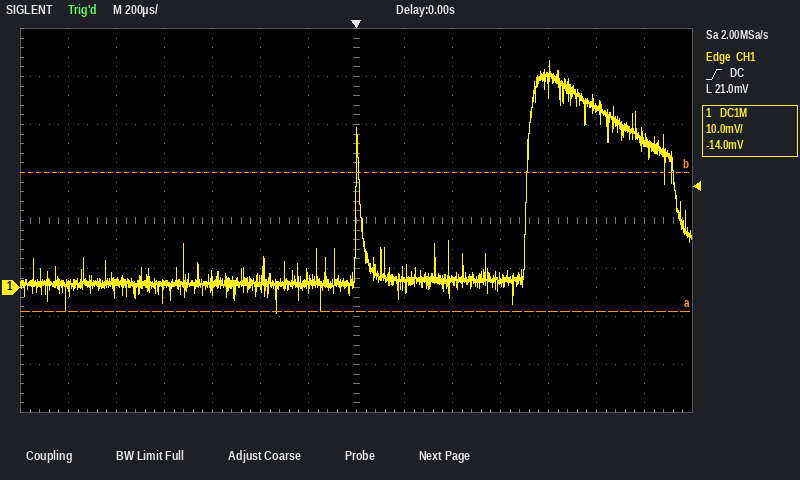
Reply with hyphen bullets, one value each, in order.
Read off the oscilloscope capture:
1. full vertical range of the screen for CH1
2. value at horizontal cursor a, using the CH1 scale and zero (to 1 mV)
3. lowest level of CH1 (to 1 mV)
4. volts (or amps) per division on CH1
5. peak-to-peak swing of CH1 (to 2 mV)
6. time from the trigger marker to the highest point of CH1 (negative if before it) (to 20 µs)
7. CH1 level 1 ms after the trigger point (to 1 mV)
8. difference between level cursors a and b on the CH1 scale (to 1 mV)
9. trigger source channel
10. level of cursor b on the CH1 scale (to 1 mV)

- 80 mV
- -5 mV
- -5 mV
- 10 mV
- 52 mV
- +800 µs
- 37 mV
- 29 mV
- CH1
- 24 mV
